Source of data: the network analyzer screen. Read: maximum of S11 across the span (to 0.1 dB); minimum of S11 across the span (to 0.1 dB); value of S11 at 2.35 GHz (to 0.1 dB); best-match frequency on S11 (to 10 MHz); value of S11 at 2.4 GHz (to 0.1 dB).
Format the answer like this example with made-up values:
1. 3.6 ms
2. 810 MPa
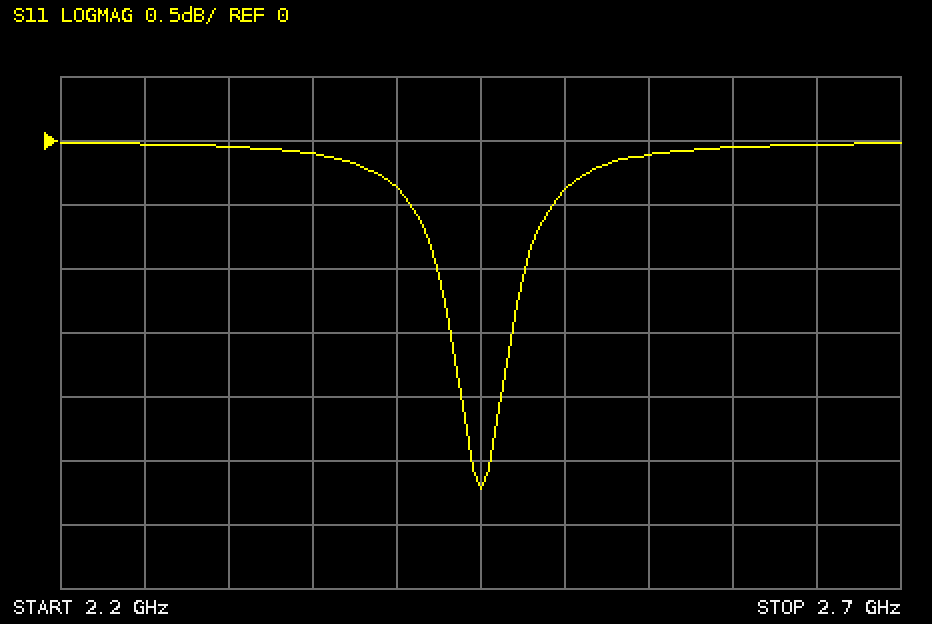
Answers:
1. 0.0 dB
2. -2.7 dB
3. -0.1 dB
4. 2.45 GHz
5. -0.4 dB
